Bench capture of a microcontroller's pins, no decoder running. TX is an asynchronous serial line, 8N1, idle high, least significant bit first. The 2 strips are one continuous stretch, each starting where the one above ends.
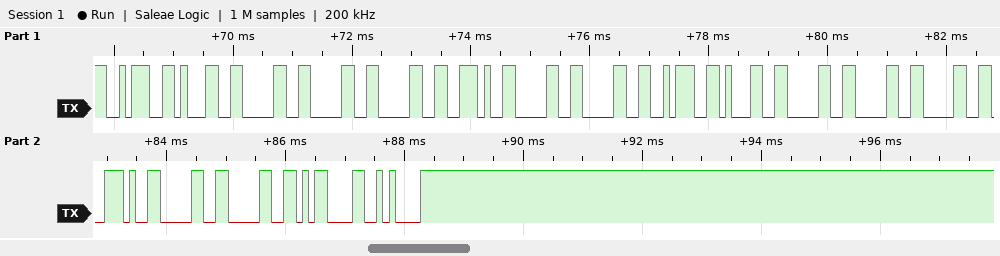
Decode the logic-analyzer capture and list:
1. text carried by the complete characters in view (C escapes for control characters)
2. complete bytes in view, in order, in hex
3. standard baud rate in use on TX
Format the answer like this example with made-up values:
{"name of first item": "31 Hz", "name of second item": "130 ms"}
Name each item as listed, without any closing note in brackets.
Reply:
{"text carried by the complete characters in view": "\":1000.00:1000.00\\r\\n\"", "complete bytes in view, in order, in hex": "3A 31 30 30 30 2E 30 30 3A 31 30 30 30 2E 30 30 0D 0A", "standard baud rate in use on TX": "9600 baud"}
